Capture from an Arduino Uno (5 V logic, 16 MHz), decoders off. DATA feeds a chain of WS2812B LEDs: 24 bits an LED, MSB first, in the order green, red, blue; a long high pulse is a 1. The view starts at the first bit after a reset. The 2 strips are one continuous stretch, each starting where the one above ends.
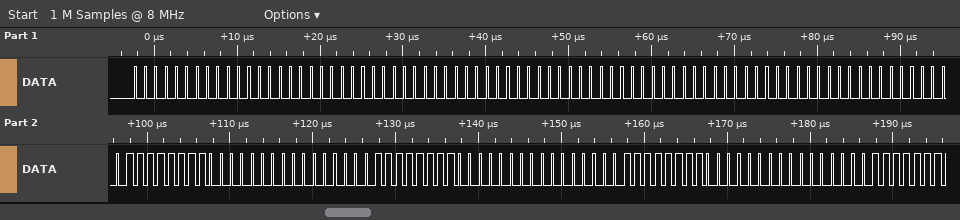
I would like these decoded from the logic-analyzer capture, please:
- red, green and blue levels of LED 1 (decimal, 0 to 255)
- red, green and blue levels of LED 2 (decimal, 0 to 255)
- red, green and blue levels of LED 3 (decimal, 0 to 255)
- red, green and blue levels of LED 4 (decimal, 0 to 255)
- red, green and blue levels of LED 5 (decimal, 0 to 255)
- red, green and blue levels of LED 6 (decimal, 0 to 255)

0, 0, 0
0, 0, 0
0, 0, 0
255, 0, 0
255, 0, 0
255, 0, 0
